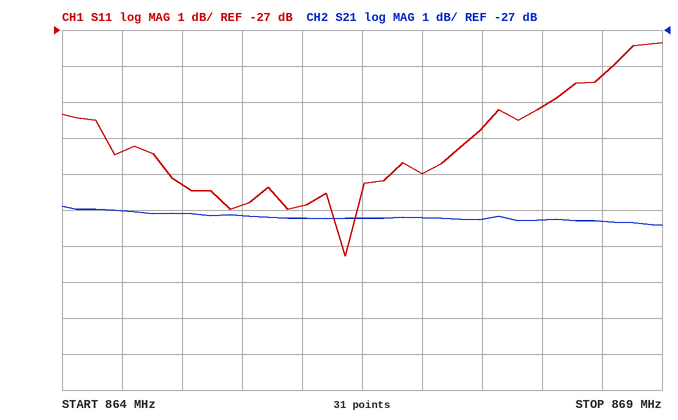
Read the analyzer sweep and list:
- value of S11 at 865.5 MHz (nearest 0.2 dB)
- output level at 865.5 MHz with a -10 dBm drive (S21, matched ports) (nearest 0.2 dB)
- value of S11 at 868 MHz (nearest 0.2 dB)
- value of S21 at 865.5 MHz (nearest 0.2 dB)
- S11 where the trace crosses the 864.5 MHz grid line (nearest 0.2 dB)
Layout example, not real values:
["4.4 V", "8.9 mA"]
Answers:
["-31.8 dB", "-42.2 dBm", "-29.2 dB", "-32.2 dB", "-30.4 dB"]
